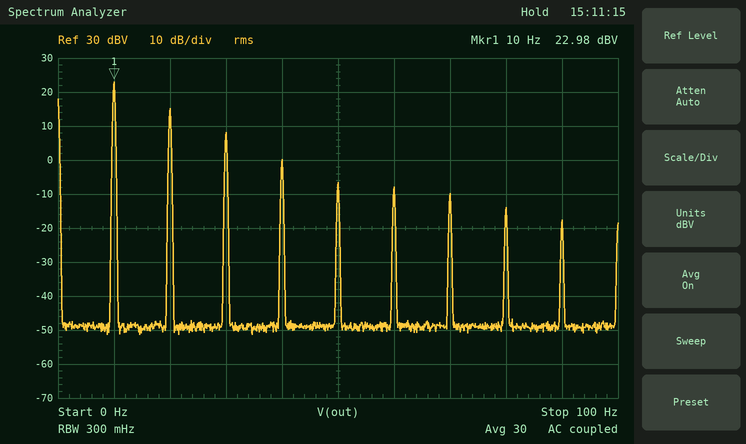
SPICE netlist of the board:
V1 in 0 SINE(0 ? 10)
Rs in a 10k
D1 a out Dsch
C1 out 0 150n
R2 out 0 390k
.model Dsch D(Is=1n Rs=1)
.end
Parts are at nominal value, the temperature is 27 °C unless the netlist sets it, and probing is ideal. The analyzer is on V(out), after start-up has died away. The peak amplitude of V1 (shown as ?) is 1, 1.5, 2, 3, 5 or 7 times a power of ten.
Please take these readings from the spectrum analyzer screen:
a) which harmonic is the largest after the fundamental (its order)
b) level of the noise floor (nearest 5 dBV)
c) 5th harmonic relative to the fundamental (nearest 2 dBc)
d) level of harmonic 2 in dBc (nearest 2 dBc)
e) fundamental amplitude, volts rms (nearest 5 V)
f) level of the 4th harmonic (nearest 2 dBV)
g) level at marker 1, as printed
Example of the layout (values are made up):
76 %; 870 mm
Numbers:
2; -50 dBV; -30 dBc; -8 dBc; 15 V; 0 dBV; 22.98 dBV
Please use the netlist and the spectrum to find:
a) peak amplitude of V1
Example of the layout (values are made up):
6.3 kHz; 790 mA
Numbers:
70 V
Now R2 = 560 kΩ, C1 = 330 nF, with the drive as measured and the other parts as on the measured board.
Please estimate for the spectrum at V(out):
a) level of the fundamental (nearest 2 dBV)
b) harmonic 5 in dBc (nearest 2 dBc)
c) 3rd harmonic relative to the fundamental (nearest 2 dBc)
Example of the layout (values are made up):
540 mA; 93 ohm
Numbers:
16 dBV; -22 dBc; -12 dBc
